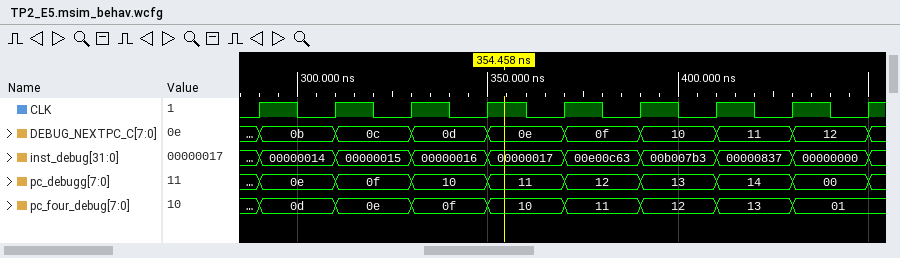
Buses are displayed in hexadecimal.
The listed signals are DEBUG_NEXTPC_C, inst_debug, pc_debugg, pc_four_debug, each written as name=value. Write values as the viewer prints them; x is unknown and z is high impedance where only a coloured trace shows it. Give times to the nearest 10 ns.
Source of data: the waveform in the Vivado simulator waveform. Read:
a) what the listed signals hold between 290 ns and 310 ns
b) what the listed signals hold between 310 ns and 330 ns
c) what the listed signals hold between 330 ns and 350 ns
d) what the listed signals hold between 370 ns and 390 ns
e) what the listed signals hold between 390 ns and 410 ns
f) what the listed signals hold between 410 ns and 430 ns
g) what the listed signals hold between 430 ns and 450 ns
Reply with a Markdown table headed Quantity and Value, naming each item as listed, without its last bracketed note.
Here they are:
| Quantity | Value |
|---|---|
| what the listed signals hold between 290 ns and 310 ns | DEBUG_NEXTPC_C=0b, inst_debug=00000014, pc_debugg=0e, pc_four_debug=0d |
| what the listed signals hold between 310 ns and 330 ns | DEBUG_NEXTPC_C=0c, inst_debug=00000015, pc_debugg=0f, pc_four_debug=0e |
| what the listed signals hold between 330 ns and 350 ns | DEBUG_NEXTPC_C=0d, inst_debug=00000016, pc_debugg=10, pc_four_debug=0f |
| what the listed signals hold between 370 ns and 390 ns | DEBUG_NEXTPC_C=0f, inst_debug=00e00c63, pc_debugg=12, pc_four_debug=11 |
| what the listed signals hold between 390 ns and 410 ns | DEBUG_NEXTPC_C=10, inst_debug=00b007b3, pc_debugg=13, pc_four_debug=12 |
| what the listed signals hold between 410 ns and 430 ns | DEBUG_NEXTPC_C=11, inst_debug=00000837, pc_debugg=14, pc_four_debug=13 |
| what the listed signals hold between 430 ns and 450 ns | DEBUG_NEXTPC_C=12, inst_debug=00000000, pc_debugg=00, pc_four_debug=01 |
